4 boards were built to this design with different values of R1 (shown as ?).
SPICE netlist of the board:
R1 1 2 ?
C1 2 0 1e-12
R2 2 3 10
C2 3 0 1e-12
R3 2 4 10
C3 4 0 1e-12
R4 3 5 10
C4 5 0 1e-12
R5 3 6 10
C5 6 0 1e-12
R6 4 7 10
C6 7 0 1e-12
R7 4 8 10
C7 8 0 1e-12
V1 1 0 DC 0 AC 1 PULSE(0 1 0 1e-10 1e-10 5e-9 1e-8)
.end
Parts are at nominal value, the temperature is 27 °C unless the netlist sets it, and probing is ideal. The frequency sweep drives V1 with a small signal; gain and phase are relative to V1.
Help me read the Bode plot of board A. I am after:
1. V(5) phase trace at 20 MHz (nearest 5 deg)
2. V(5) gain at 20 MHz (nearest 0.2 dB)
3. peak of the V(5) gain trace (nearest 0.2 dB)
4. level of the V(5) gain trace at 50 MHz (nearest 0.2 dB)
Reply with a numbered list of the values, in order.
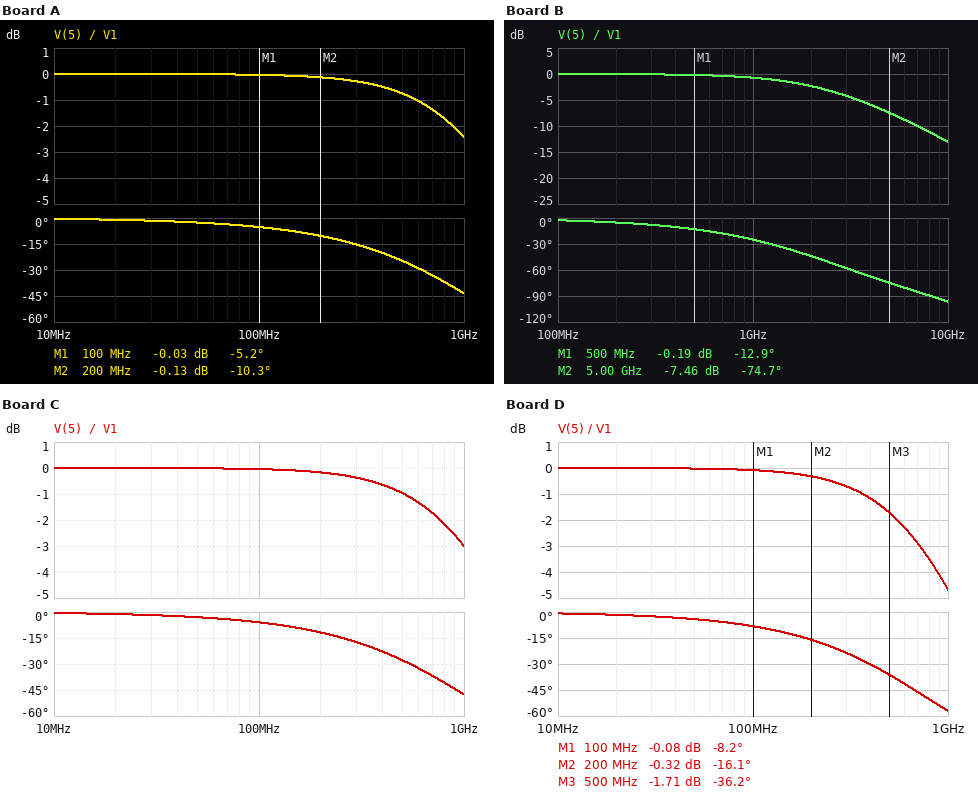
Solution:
1. 0 deg
2. 0 dB
3. 0 dB
4. 0 dB
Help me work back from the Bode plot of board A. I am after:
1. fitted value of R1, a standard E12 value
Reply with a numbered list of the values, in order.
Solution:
1. 15 Ω
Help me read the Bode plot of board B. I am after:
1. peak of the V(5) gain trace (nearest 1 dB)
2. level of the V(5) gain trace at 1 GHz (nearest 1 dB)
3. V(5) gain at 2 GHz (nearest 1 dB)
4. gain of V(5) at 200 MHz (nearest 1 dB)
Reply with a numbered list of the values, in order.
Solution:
1. 0 dB
2. -1 dB
3. -2 dB
4. 0 dB
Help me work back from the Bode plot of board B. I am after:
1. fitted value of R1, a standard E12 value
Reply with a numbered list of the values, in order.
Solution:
1. 4.7 Ω
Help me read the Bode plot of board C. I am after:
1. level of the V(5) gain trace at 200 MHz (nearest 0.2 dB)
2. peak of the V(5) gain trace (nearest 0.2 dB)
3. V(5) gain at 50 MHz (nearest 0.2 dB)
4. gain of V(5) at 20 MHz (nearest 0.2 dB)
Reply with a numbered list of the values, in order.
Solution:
1. -0.2 dB
2. 0 dB
3. 0 dB
4. 0 dB
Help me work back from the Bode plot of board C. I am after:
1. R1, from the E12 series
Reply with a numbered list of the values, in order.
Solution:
1. 18 Ω
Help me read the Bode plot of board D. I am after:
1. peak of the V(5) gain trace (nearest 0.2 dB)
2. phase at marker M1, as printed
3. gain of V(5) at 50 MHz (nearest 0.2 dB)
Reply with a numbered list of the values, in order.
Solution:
1. 0 dB
2. -8.2 deg
3. 0 dB
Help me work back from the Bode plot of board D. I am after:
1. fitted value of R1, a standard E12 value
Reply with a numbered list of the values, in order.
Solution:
1. 27 Ω
